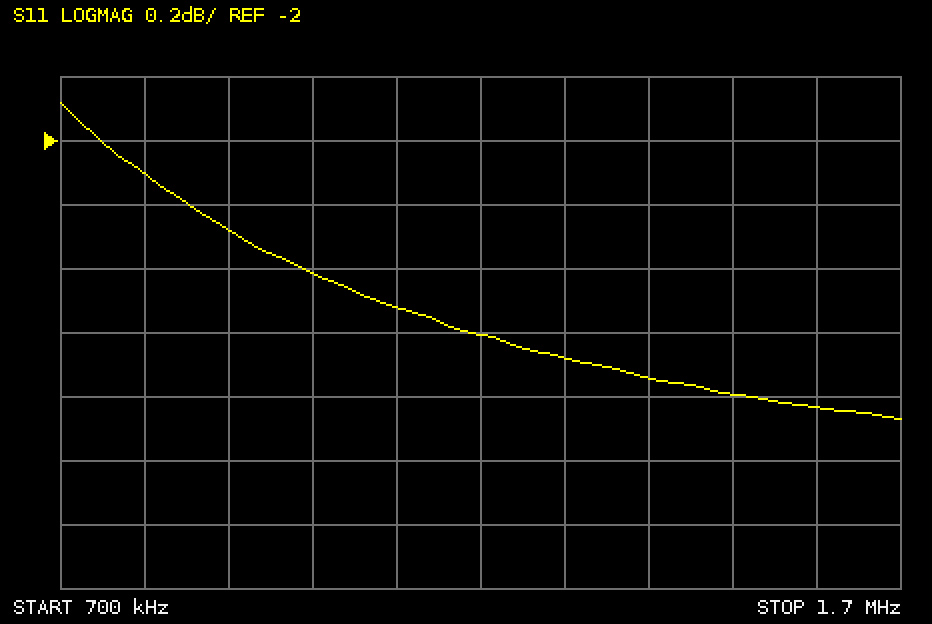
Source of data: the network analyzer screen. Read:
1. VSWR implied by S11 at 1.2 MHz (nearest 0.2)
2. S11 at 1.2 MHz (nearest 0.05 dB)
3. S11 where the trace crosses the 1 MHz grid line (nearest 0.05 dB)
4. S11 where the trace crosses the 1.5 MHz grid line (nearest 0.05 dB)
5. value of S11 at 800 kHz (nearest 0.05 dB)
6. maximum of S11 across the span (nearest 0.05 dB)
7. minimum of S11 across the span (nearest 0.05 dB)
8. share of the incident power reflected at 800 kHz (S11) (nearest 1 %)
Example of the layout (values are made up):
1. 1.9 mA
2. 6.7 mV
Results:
1. 6.8
2. -2.60 dB
3. -2.40 dB
4. -2.80 dB
5. -2.10 dB
6. -1.90 dB
7. -2.85 dB
8. 62 %
